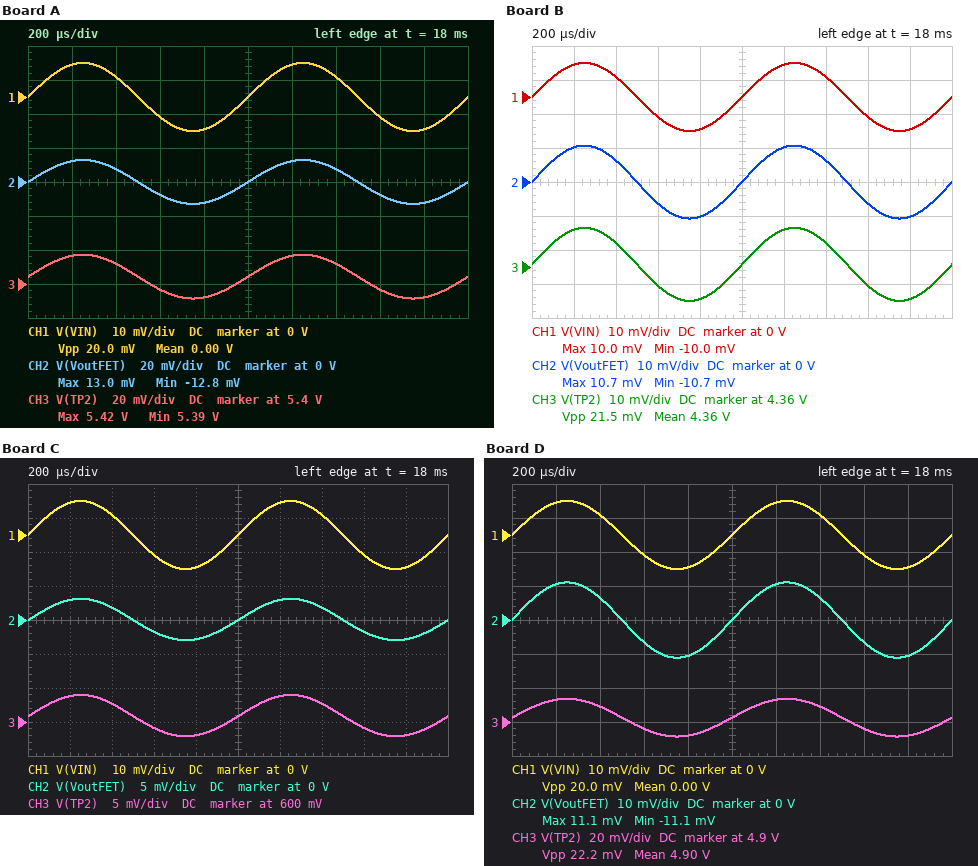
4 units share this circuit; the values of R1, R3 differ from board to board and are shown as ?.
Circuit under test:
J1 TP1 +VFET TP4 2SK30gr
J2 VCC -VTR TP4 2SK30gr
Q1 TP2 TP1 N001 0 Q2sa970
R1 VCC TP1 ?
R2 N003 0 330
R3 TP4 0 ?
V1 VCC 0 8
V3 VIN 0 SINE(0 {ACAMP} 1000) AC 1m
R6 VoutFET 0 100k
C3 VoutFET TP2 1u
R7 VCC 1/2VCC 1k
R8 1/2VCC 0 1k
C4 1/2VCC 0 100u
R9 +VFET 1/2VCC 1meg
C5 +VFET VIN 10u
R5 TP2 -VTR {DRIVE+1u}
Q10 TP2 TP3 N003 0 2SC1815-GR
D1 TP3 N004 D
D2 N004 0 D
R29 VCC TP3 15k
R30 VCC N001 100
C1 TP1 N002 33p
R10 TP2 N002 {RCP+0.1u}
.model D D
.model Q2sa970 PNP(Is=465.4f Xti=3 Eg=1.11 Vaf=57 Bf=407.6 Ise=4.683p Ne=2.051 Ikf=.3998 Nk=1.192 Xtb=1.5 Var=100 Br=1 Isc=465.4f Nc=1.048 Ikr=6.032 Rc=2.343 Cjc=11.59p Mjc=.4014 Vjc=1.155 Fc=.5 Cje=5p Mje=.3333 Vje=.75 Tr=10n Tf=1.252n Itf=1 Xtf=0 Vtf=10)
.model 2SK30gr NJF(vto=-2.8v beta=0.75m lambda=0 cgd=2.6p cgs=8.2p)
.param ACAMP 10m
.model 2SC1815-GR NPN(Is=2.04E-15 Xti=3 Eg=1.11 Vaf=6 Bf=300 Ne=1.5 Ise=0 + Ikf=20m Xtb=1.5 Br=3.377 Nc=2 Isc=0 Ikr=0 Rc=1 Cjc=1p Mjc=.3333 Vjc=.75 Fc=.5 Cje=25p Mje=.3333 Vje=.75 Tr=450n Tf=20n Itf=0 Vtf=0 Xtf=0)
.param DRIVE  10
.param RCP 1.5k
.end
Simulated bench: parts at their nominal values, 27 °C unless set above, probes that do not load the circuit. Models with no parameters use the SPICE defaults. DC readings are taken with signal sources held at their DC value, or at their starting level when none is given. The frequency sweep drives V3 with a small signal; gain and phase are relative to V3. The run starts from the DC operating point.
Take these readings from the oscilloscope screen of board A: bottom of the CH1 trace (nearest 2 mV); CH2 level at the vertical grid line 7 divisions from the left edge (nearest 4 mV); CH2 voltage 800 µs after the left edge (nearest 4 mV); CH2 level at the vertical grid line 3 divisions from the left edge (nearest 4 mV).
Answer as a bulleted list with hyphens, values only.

- -10 mV
- 8 mV
- -12 mV
- -8 mV
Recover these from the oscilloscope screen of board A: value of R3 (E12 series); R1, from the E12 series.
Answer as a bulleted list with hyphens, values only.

- 2.7 kΩ
- 8.2 kΩ
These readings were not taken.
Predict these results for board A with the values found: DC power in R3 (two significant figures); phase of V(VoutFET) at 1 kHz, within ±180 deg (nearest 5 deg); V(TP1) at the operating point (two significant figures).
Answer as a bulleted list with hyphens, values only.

- 15 mW
- 0 deg
- 7.3 V
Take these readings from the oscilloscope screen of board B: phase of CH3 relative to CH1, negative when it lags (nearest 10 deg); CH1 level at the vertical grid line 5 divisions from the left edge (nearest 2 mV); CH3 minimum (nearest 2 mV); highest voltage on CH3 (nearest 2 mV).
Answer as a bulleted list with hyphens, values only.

- 0 deg
- 0 V
- 4.350 V
- 4.372 V
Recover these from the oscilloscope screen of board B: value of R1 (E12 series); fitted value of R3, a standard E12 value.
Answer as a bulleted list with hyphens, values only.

- 6.8 kΩ
- 12 kΩ
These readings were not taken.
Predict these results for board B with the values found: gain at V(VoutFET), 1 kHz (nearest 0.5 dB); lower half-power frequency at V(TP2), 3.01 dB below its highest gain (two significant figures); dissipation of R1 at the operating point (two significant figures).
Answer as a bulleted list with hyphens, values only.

- 0.5 dB
- 16 mHz
- 81 µW
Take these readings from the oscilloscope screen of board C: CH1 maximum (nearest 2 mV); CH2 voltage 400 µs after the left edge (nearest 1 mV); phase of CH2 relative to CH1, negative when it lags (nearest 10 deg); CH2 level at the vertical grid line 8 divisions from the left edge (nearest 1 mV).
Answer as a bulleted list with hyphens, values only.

- 10 mV
- 2 mV
- 0 deg
- -2 mV
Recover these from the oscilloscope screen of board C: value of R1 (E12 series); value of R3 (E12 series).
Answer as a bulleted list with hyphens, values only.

- 1.8 kΩ
- 15 kΩ
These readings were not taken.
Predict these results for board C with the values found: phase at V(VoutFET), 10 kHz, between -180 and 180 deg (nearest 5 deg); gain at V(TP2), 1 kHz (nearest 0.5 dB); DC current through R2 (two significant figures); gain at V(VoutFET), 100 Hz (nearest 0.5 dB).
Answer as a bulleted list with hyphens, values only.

- -5 deg
- -10.5 dB
- 1.6 mA
- -10.5 dB
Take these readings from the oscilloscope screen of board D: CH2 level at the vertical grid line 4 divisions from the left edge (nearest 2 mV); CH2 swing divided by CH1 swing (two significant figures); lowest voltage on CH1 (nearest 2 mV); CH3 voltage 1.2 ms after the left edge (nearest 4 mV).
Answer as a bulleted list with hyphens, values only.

- -10 mV
- 1.1
- -10 mV
- 4.912 V
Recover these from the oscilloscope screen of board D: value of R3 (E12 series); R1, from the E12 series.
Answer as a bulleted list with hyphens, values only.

- 4.7 kΩ
- 6.8 kΩ
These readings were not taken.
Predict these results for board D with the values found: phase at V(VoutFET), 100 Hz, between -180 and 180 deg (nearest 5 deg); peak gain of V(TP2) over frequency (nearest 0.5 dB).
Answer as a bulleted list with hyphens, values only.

- 0 deg
- 1.0 dB
